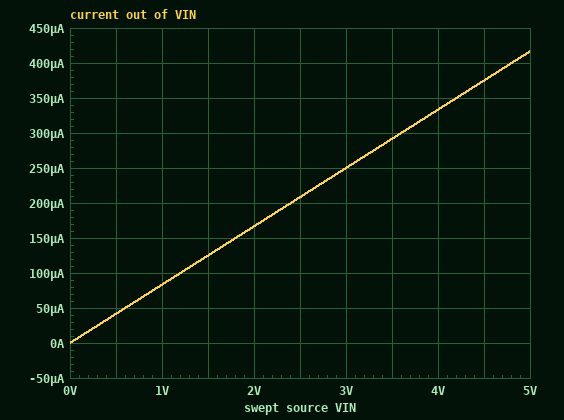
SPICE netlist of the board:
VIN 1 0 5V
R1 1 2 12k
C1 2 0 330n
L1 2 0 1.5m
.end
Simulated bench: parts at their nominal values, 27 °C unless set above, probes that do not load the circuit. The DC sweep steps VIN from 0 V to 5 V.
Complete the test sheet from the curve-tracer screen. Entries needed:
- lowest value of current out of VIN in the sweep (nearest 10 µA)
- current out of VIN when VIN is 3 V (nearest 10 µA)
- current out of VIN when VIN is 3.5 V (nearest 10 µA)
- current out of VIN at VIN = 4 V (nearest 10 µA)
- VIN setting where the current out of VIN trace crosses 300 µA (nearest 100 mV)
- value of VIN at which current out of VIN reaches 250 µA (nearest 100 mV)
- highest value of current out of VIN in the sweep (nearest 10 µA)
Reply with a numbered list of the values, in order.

1. 0 A
2. 250 µA
3. 290 µA
4. 330 µA
5. 3.6 V
6. 3.0 V
7. 420 µA
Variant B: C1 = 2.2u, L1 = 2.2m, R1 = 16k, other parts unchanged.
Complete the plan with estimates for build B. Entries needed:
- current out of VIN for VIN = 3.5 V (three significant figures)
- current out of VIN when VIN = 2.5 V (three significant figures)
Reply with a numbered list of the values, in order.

1. 219 µA
2. 156 µA
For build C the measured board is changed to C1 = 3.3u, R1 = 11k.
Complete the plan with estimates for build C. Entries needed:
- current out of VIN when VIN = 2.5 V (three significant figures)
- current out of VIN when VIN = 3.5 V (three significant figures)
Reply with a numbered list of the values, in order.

1. 227 µA
2. 318 µA
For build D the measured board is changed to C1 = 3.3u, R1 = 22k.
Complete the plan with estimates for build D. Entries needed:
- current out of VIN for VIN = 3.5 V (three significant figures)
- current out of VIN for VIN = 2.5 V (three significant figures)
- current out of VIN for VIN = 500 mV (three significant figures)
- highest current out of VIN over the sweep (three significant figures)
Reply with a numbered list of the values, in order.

1. 159 µA
2. 114 µA
3. 22.7 µA
4. 227 µA
